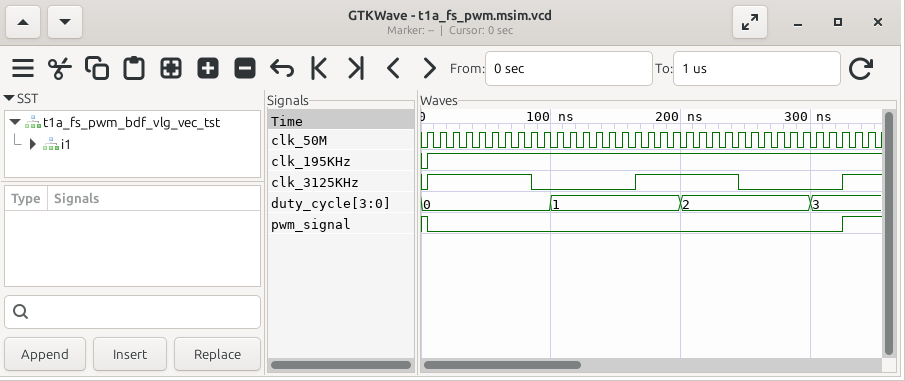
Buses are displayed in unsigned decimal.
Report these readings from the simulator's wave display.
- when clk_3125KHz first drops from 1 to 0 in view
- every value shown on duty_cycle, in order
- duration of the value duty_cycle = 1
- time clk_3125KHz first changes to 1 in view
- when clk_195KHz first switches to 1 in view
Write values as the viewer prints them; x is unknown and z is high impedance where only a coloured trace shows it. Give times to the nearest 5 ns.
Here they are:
85 ns
0, 1, 2, 3
100 ns
5 ns
5 ns
